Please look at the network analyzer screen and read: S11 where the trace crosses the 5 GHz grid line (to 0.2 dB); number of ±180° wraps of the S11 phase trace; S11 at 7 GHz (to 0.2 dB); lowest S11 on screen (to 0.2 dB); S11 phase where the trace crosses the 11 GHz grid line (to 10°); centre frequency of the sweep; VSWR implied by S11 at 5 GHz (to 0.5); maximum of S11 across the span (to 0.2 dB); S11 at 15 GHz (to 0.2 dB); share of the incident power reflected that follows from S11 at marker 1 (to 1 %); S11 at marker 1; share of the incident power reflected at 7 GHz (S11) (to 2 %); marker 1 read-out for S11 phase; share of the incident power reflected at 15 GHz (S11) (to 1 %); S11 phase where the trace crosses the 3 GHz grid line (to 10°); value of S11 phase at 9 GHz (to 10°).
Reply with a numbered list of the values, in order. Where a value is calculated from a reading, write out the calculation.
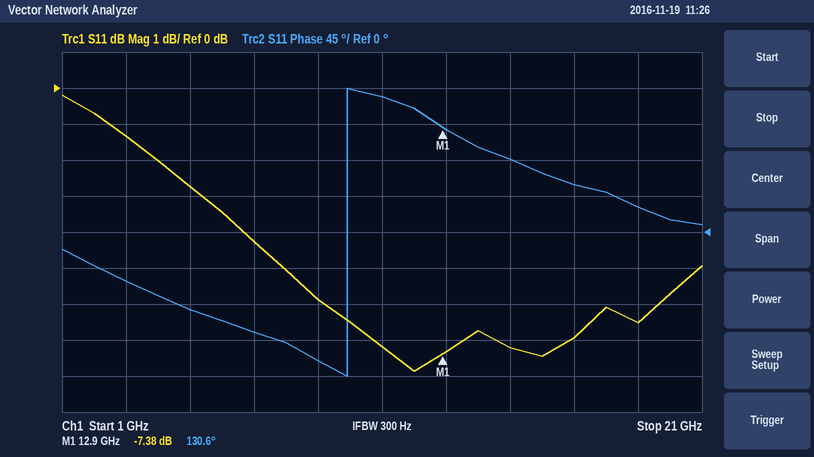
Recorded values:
1. -2.8 dB
2. 1
3. -4.2 dB
4. -7.8 dB
5. 170°
6. 11 GHz
7. |Γ| = 10^(-2.8/20) = 0.7244; VSWR = (1 + 0.7244)/(1 − 0.7244) ≈ 6.26, so 6.5 to the nearest 0.5
8. -0.2 dB
9. -7.2 dB
10. 10^(-7.38/10) ≈ 18 %
11. -7.38 dB
12. 10^(-4.2/10) ≈ 38 %
13. 130.6°
14. 10^(-7.2/10) ≈ 19 %
15. -60°
16. -160°
